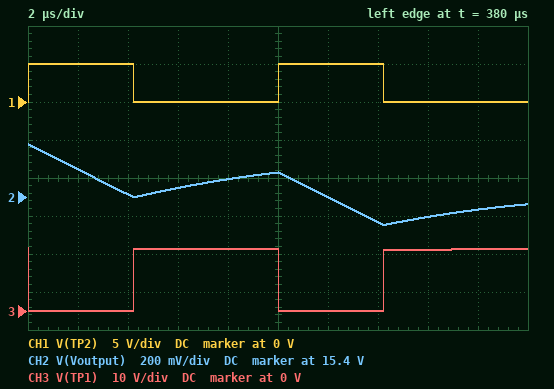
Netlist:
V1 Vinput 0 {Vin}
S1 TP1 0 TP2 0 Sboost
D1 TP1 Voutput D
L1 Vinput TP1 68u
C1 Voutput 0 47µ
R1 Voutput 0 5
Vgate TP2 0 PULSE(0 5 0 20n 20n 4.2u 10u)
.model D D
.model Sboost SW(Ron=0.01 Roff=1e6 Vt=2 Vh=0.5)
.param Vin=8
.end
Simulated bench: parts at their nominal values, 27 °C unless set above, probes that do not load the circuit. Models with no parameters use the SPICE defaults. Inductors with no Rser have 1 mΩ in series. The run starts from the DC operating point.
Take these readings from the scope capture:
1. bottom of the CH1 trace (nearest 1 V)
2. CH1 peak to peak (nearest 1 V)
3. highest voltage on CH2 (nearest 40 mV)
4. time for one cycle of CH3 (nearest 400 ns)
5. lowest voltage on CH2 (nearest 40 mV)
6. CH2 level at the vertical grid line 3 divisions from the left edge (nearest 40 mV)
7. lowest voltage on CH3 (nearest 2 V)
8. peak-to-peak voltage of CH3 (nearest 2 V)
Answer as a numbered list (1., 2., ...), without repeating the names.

1. 0 V
2. 5 V
3. 15.68 V
4. 10.0 µs
5. 15.24 V
6. 15.44 V
7. 0 V
8. 16 V
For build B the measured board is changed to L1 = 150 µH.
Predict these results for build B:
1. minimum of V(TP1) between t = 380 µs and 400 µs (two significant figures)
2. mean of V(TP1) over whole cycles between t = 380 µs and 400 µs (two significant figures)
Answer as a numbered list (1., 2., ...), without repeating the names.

1. 60 mV
2. 8.7 V
